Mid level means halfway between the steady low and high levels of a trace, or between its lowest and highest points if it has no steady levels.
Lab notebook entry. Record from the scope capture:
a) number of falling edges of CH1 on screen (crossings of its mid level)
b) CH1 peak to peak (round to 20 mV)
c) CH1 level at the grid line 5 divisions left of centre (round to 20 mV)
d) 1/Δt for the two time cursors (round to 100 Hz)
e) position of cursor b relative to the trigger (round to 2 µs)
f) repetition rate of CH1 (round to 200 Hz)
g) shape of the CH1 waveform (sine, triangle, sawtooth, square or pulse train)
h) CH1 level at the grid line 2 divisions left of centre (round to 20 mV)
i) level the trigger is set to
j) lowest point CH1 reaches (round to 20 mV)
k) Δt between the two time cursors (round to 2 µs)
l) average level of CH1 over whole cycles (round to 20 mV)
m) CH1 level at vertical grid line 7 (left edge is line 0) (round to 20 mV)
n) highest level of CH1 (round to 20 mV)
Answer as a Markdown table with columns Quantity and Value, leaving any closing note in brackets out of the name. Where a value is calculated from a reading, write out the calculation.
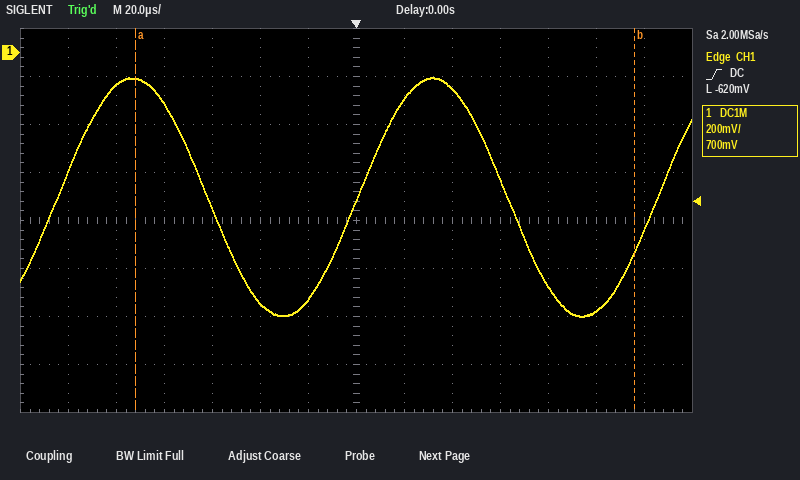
| Quantity | Value |
|---|---|
| number of falling edges of CH1 on screen | 2 |
| CH1 peak to peak | -100 mV − (-1.10 V) = 1.00 V |
| CH1 level at the grid line 5 divisions left of centre | -140 mV |
| 1/Δt for the two time cursors | 1 / 208 µs ≈ 4.8 kHz |
| position of cursor b relative to the trigger | +116 µs |
| repetition rate of CH1 | 8.0 kHz |
| shape of the CH1 waveform | sine |
| CH1 level at the grid line 2 divisions left of centre | -1.04 V |
| level the trigger is set to | -620 mV |
| lowest point CH1 reaches | -1.10 V |
| Δt between the two time cursors | 208 µs |
| average level of CH1 over whole cycles | (-100 mV + (-1.10 V)) / 2 ≈ -600 mV |
| CH1 level at vertical grid line 7 (left edge is line 0) | -620 mV |
| highest level of CH1 | -100 mV |
